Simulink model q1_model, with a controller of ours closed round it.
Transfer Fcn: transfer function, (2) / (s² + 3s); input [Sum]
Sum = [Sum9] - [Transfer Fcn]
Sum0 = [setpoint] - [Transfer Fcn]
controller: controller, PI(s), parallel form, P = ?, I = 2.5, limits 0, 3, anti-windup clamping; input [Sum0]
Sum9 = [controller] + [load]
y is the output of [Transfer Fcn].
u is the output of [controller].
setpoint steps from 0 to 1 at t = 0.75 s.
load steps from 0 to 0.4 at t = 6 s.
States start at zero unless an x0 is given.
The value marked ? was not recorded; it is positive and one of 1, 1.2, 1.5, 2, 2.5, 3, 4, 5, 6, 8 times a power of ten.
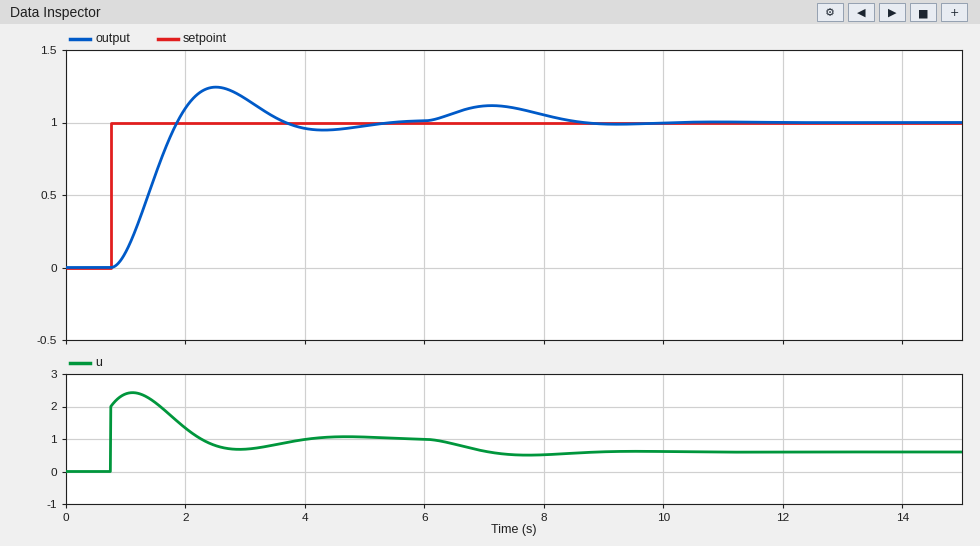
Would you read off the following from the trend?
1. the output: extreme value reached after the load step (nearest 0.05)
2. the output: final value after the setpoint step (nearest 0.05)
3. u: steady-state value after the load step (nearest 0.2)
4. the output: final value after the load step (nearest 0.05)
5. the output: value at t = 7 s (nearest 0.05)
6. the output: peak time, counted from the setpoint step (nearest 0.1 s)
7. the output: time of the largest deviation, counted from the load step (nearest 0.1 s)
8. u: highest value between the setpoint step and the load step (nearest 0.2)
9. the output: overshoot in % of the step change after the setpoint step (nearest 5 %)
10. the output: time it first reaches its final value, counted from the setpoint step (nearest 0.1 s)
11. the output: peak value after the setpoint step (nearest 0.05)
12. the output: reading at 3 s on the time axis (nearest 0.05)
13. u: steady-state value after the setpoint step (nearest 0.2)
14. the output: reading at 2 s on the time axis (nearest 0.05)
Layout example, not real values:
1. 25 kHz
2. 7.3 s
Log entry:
1. 1.10
2. 1.00
3. 0.6
4. 1.00
5. 1.10
6. 1.8 s
7. 1.1 s
8. 2.4
9. 25 %
10. 1.1 s
11. 1.25
12. 1.15
13. 1.0
14. 1.10
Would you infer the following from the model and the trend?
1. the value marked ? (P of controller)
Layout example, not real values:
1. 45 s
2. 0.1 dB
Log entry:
1. 2
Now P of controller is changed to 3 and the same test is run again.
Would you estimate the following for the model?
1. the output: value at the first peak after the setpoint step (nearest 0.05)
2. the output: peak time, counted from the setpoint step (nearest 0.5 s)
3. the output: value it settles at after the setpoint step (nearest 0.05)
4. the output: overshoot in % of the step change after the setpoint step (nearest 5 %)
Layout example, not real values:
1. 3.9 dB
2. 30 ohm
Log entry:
1. 1.15
2. 1.5 s
3. 1.00
4. 15 %
